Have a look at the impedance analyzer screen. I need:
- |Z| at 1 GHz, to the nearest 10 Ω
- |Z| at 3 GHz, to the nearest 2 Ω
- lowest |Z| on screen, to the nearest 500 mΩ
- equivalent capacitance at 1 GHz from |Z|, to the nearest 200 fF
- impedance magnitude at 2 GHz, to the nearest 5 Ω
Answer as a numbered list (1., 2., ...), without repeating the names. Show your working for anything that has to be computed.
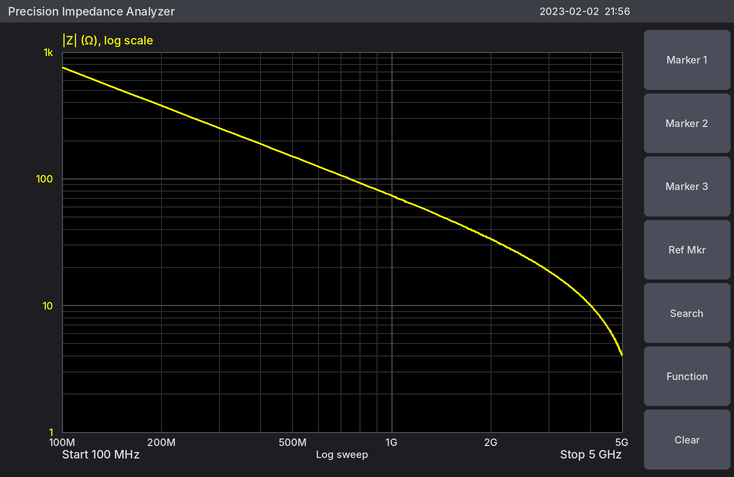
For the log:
1. 70 Ω
2. 18 Ω
3. 4.0 Ω
4. C = 1/(2π × 1 GHz × 70 Ω) ≈ 2.27 pF, so 2.2 pF to the nearest 200 fF
5. 35 Ω
